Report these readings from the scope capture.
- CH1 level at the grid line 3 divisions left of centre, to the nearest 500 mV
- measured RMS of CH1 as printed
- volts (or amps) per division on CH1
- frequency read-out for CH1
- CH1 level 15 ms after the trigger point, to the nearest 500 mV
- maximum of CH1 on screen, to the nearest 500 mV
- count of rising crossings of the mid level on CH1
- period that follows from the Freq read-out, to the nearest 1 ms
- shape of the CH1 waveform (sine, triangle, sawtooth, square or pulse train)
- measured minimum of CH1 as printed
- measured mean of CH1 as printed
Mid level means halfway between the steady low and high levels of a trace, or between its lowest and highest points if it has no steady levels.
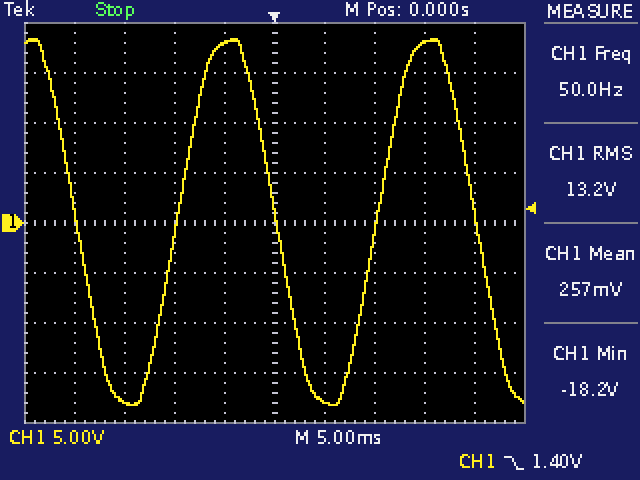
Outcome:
-18.0 V
13.2 V
5 V
50.0 Hz
18.0 V
18.5 V
2
20 ms
sine
-18.2 V
257 mV
